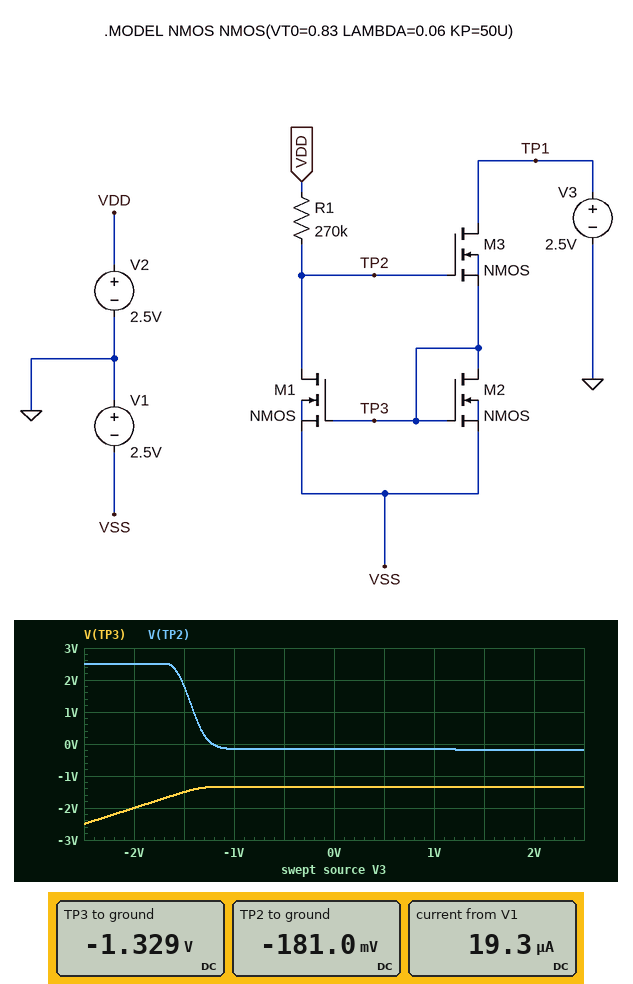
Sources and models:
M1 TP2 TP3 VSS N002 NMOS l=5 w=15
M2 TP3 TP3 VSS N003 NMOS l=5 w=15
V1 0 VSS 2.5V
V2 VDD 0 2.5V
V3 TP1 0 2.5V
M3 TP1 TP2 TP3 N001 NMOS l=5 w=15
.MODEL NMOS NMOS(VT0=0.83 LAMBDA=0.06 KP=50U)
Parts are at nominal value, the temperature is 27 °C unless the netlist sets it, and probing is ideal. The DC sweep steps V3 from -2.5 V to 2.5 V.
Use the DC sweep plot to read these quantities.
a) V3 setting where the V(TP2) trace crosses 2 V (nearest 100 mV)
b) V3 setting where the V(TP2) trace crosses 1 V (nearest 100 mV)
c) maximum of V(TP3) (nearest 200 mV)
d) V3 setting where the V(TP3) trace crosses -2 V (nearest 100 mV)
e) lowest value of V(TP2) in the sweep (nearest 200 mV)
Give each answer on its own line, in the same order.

-1.5 V
-1.4 V
-1.4 V
-2.0 V
-200 mV
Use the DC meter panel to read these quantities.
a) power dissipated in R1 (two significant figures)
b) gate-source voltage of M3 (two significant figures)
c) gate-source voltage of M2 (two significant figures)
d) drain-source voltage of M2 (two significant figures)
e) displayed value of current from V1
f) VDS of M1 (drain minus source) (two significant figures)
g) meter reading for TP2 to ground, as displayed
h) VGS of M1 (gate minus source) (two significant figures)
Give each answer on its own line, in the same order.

27 µW
1.1 V
1.2 V
1.2 V
19.3 µA
2.3 V
-181.0 mV
1.2 V
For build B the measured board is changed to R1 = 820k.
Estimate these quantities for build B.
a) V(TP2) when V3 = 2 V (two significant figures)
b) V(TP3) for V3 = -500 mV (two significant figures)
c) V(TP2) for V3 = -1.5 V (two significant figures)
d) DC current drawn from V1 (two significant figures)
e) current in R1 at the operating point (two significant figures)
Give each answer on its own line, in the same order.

-440 mV
-1.5 V
640 mV
7.0 µA
3.6 µA
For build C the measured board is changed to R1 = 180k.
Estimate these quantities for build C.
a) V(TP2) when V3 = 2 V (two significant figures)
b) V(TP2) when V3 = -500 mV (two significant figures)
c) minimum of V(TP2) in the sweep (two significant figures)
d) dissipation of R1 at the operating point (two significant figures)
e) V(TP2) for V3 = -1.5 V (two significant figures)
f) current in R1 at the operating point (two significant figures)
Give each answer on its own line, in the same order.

-50 mV
-27 mV
-54 mV
36 µW
2.0 V
14 µA
